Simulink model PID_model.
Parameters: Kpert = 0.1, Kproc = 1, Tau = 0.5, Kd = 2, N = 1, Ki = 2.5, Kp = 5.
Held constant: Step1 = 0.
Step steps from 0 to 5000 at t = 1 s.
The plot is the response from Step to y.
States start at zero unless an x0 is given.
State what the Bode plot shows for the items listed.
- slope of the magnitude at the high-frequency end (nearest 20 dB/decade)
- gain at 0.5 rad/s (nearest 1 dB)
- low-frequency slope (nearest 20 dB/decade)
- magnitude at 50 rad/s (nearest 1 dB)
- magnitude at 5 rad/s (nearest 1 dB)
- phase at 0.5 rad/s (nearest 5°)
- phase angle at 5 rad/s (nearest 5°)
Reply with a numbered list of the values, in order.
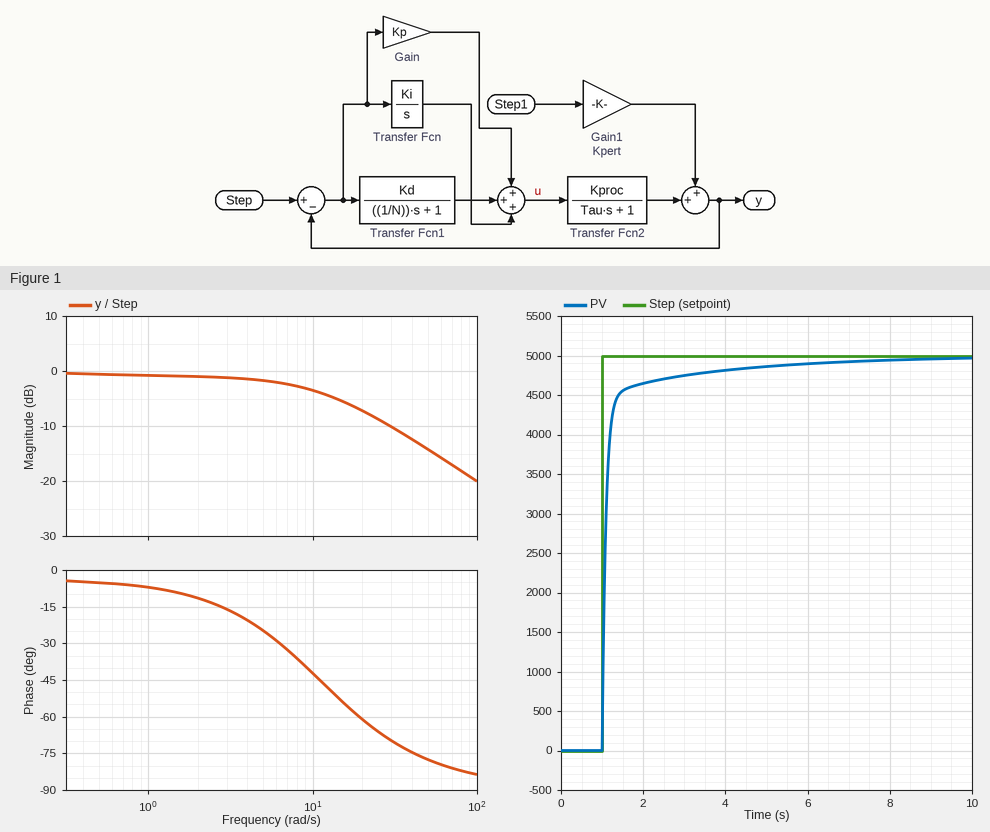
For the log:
1. -20 dB/decade
2. -1 dB
3. 0 dB/decade
4. -14 dB
5. -2 dB
6. -5°
7. -25°
